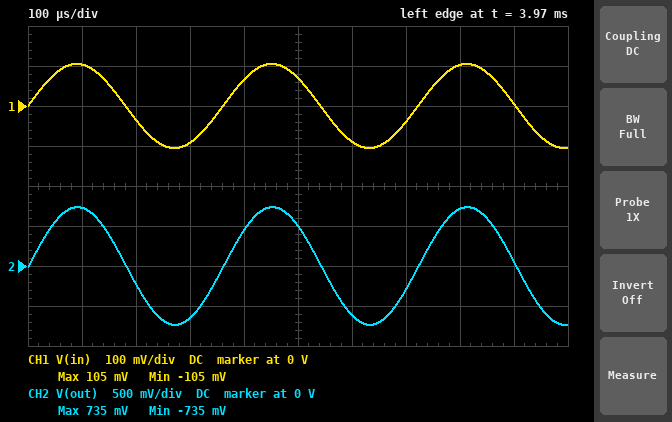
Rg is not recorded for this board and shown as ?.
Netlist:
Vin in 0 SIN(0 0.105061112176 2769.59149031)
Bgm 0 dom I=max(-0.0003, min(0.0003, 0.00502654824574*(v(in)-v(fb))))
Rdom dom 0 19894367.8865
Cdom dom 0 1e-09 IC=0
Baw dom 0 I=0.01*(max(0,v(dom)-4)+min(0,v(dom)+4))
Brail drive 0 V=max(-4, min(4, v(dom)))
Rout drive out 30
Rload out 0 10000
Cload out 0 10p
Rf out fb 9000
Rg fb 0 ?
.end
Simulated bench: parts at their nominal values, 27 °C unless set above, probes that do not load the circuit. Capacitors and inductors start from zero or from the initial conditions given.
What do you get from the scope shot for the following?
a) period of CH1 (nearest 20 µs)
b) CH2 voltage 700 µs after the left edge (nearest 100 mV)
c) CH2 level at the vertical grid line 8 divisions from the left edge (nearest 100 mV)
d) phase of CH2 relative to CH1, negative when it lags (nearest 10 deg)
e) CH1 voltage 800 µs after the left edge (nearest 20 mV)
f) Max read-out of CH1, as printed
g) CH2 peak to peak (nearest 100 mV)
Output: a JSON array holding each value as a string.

["360 µs", "-300 mV", "700 mV", "0 deg", "100 mV", "105 mV", "1.5 V"]
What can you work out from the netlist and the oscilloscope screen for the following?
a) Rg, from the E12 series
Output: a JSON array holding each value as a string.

["1.5 kΩ"]
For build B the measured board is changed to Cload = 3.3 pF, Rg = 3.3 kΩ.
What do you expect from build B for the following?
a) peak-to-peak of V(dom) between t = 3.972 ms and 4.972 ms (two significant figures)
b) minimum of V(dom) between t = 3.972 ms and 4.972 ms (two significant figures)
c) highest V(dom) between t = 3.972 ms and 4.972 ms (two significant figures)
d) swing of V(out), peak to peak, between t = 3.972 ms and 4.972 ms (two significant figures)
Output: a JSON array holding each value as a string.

["790 mV", "-390 mV", "390 mV", "780 mV"]
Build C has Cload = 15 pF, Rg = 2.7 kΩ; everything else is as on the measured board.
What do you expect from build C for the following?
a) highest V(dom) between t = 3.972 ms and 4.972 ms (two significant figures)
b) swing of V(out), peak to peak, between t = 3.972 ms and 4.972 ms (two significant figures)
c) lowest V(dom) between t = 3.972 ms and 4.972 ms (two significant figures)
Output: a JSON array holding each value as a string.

["460 mV", "910 mV", "-460 mV"]
